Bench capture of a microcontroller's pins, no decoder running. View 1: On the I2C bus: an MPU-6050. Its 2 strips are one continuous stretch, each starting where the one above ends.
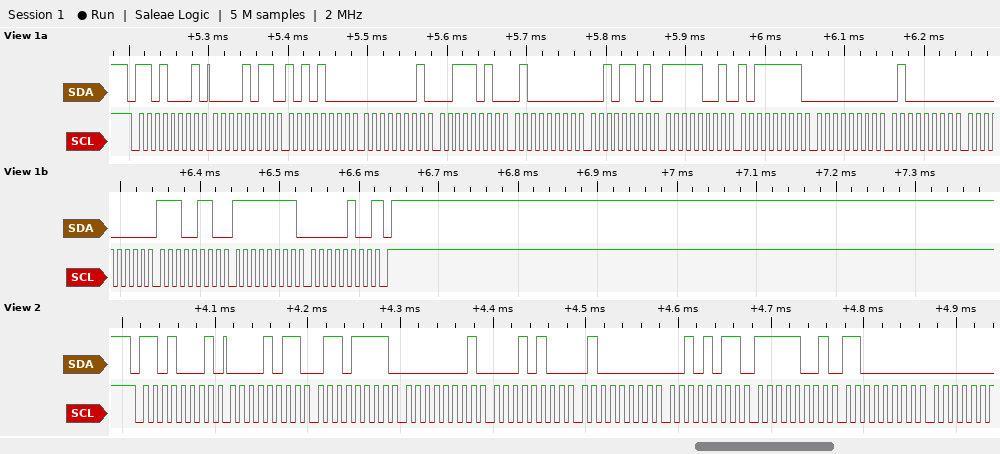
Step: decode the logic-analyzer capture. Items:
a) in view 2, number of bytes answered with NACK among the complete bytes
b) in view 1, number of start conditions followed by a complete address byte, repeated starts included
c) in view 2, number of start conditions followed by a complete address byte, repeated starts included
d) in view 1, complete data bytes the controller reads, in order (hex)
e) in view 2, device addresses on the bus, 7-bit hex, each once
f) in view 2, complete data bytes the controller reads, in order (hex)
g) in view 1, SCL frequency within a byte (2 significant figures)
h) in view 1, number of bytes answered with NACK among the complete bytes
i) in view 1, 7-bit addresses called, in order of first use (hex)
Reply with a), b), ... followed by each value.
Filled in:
a) 0
b) 1
c) 1
d) 0B A8 01 3A 40 2D F9 BF 00 40 00 E6 FF 04
e) 0x68
f) 0B 6F 01 14 40 2B F9 C0
g) 100 kHz
h) 1
i) 0x68
